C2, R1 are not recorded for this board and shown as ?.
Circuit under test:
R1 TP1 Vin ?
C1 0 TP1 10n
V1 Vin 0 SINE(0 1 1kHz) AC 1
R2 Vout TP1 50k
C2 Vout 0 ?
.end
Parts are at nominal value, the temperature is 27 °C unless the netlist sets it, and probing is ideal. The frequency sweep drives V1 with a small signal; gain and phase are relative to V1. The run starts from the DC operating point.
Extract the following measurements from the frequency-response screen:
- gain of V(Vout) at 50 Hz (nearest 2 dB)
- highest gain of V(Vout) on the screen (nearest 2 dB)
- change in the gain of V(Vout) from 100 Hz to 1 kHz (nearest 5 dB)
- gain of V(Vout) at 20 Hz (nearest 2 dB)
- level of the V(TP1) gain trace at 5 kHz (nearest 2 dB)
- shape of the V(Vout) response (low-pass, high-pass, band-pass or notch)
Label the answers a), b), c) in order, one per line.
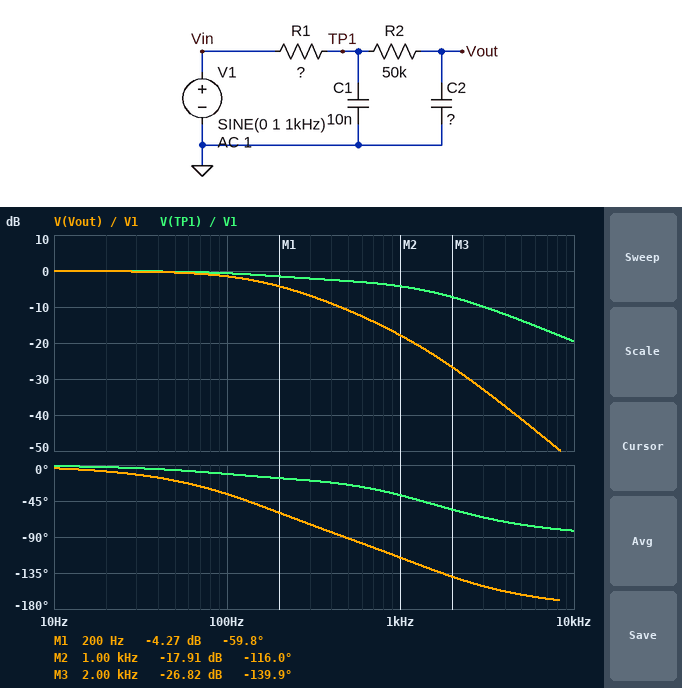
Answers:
a) 0 dB
b) 0 dB
c) -15 dB
d) 0 dB
e) -14 dB
f) low-pass
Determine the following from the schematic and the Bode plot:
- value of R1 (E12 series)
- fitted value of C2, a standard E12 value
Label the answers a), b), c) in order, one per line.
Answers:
a) 15 kΩ
b) 15 nF
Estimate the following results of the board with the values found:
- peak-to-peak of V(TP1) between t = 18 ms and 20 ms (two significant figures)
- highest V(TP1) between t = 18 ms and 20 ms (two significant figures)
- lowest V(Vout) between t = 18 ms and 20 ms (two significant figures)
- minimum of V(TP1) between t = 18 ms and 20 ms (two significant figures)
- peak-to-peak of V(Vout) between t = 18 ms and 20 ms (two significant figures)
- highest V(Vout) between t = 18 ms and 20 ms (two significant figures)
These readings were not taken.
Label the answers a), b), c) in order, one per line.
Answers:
a) 1.2 V
b) 610 mV
c) -130 mV
d) -610 mV
e) 250 mV
f) 130 mV
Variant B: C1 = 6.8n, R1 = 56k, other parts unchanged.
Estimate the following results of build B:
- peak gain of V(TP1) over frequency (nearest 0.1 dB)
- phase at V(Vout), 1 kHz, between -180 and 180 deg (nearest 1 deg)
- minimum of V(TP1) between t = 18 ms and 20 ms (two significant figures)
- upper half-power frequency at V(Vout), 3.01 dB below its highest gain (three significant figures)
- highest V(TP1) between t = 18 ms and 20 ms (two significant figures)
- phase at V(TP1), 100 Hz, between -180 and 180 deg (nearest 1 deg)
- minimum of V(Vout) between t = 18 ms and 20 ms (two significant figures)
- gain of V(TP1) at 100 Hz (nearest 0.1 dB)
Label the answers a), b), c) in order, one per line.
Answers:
a) 0 dB
b) -130 deg
c) -300 mV
d) 87.1 Hz
e) 300 mV
f) -29 deg
g) -62 mV
h) -2.8 dB
